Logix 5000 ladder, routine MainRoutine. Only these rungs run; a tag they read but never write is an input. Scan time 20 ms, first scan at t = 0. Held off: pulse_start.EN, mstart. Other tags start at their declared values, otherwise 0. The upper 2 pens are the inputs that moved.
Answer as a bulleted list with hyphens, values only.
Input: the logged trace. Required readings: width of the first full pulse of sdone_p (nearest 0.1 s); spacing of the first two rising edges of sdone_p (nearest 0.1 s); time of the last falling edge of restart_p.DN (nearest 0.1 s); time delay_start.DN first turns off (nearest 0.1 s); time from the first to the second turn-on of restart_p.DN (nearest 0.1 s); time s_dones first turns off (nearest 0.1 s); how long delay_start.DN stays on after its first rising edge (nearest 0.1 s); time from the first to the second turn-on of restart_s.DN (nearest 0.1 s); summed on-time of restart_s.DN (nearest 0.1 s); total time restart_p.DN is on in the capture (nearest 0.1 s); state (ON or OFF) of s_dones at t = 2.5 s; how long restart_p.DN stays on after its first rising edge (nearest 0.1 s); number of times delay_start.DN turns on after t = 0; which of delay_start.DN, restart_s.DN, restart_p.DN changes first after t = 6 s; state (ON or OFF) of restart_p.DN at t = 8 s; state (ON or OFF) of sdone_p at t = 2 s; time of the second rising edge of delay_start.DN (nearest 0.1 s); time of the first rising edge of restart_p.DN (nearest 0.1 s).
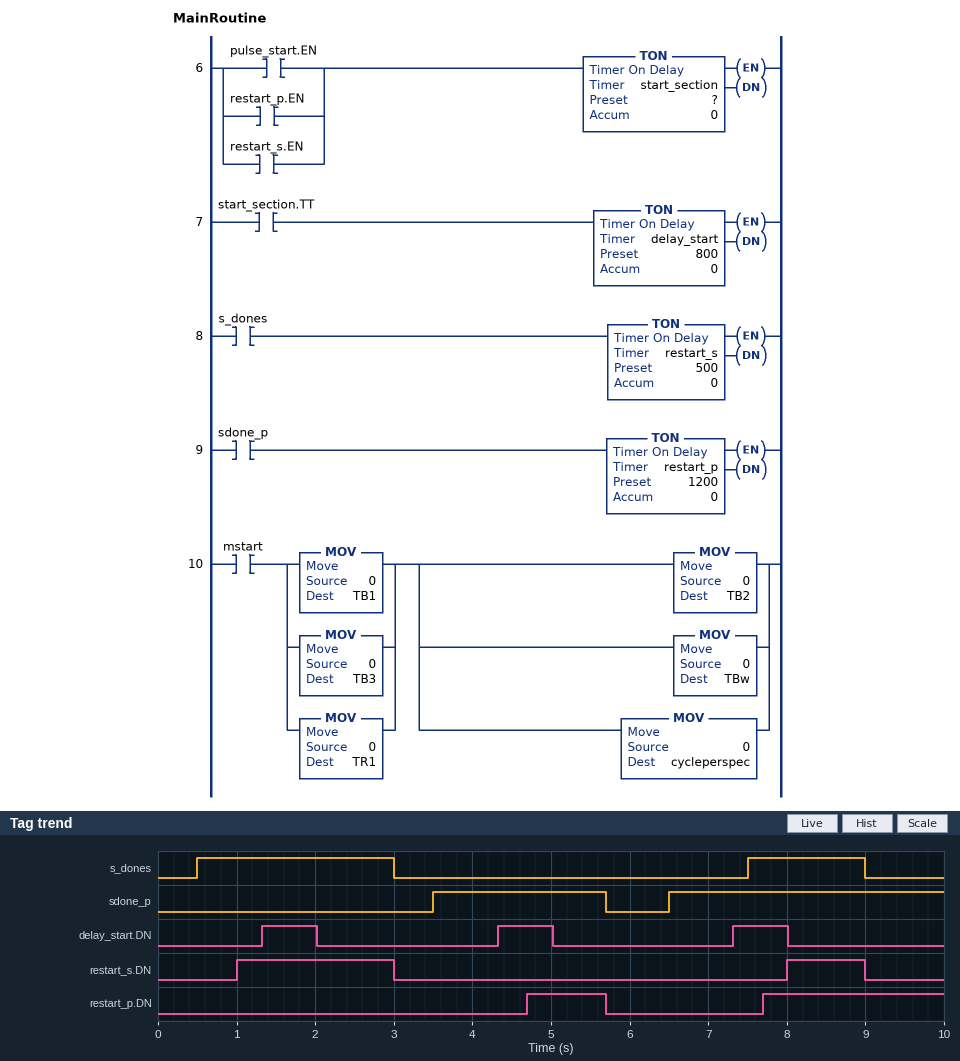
- 2.2 s
- 3.0 s
- 5.7 s
- 2.0 s
- 3.0 s
- 3.0 s
- 0.7 s
- 7.0 s
- 3.0 s
- 3.3 s
- ON
- 1.0 s
- 3
- delay_start.DN
- ON
- OFF
- 4.3 s
- 4.7 s
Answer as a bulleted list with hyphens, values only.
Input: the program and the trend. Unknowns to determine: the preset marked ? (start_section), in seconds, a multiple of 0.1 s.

- 1.5 s
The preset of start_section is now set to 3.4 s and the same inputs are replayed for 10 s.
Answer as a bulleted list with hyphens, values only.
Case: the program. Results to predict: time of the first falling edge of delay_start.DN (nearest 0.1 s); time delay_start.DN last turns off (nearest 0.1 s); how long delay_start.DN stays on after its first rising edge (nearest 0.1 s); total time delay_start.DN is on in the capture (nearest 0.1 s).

- 3.0 s
- 9.9 s
- 1.7 s
- 5.7 s
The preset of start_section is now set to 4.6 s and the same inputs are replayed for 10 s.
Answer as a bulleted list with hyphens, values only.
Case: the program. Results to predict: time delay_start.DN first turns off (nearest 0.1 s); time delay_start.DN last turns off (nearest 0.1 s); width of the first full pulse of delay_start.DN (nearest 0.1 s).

- 3.0 s
- 5.7 s
- 1.7 s
